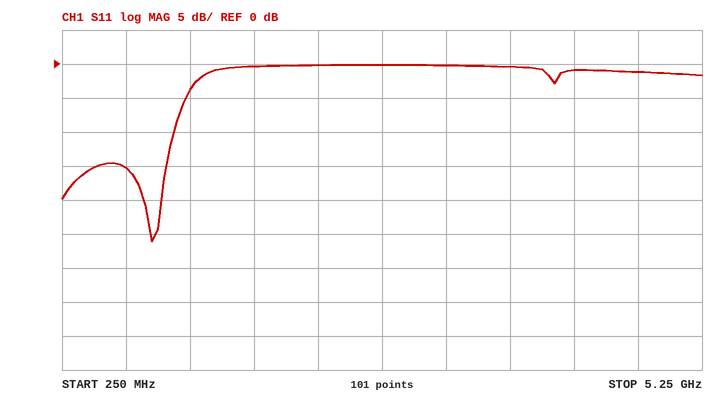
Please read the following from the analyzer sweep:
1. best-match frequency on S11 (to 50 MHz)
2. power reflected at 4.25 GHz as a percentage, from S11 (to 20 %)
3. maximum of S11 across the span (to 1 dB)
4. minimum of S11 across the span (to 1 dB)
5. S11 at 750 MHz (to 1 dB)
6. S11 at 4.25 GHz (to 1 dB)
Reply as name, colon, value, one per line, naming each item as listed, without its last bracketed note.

best-match frequency on S11: 950 MHz
power reflected at 4.25 GHz as a percentage, from S11: 80 %
maximum of S11 across the span: 0 dB
minimum of S11 across the span: -26 dB
S11 at 750 MHz: -15 dB
S11 at 4.25 GHz: -1 dB
